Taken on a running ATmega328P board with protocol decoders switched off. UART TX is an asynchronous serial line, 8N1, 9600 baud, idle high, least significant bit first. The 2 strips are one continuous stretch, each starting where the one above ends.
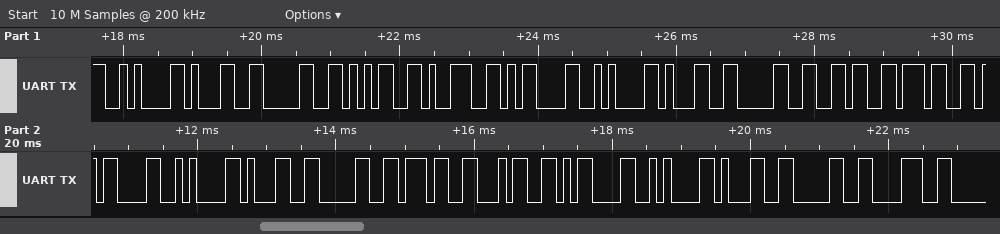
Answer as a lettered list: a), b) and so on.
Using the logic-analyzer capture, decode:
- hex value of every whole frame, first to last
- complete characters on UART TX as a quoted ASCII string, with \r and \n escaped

a) 0A 31 30 35 39 0D 0A 31 30 36 37 0D 0A 31 30 37 34 0D 0A 31 30 38
b) "\n1059\r\n1067\r\n1074\r\n108"
